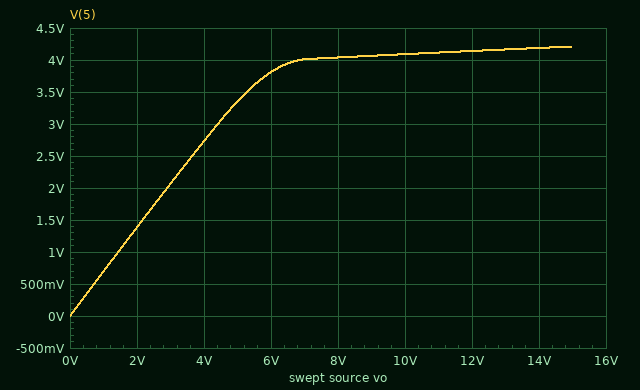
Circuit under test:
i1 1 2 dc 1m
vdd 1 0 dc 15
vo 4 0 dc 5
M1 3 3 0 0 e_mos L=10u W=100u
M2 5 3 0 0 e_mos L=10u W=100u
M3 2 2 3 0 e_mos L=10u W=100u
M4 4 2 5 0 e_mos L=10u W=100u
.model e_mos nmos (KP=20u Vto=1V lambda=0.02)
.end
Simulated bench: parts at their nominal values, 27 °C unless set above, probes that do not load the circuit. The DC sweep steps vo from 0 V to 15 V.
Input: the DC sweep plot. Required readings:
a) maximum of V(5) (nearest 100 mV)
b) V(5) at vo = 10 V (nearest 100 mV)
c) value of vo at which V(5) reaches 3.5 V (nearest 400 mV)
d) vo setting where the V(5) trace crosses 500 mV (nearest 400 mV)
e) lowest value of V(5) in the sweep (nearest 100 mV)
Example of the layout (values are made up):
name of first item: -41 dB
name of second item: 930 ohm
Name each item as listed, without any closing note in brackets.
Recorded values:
maximum of V(5): 4.2 V
V(5) at vo = 10 V: 4.1 V
value of vo at which V(5) reaches 3.5 V: 5.2 V
vo setting where the V(5) trace crosses 500 mV: 800 mV
lowest value of V(5) in the sweep: 0 V
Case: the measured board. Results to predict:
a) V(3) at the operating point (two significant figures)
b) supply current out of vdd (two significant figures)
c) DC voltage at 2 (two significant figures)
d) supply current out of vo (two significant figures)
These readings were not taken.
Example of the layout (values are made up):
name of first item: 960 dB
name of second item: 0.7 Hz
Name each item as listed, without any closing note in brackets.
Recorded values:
V(3) at the operating point: 4.0 V
supply current out of vdd: 1.0 mA
DC voltage at 2: 8.1 V
supply current out of vo: 990 µA
